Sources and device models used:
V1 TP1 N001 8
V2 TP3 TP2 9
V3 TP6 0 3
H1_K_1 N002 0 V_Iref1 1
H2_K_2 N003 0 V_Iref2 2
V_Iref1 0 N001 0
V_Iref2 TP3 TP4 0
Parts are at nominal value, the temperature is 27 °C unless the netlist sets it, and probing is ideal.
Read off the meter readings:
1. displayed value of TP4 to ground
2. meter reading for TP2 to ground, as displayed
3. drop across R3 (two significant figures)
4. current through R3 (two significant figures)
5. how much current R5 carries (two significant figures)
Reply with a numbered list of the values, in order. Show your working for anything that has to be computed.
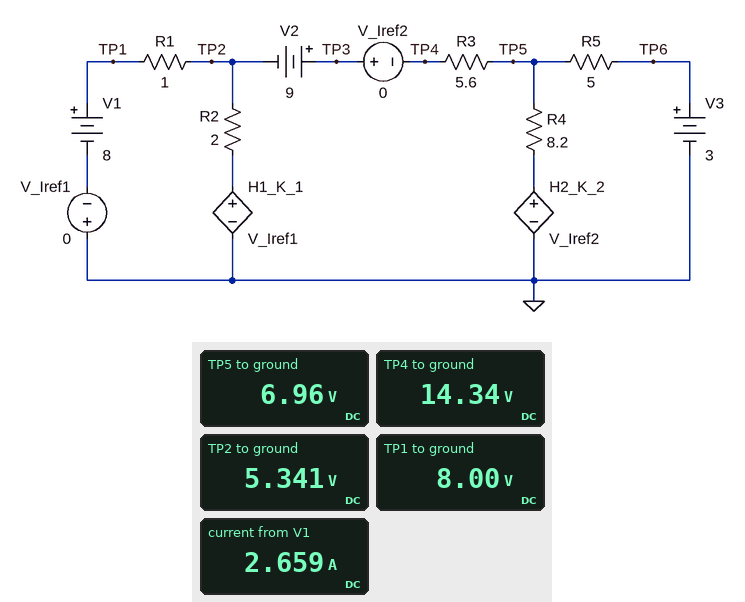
1. 14.34 V
2. 5.341 V
3. 14.34 V - 6.96 V = 7.4 V
4. (14.34 V - 6.96 V) / 5.6 Ω = 1.3 A
5. (6.96 V - 3 V) / 5 Ω = 790 mA
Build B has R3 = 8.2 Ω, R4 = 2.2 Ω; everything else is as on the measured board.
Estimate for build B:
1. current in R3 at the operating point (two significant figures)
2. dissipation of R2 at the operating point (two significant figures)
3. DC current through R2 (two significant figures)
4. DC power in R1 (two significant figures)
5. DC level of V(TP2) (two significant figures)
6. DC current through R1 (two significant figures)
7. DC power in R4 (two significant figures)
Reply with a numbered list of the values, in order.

1. 1.2 A
2. 3.9 W
3. 1.4 A
4. 6.8 W
5. 5.4 V
6. 2.6 A
7. 1.9 W
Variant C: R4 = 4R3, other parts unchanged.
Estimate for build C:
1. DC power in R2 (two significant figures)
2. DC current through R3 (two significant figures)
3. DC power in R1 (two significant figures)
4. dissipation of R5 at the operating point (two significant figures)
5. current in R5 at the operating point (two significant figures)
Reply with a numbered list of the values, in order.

1. 3.3 W
2. 1.4 A
3. 7.4 W
4. 2.1 W
5. 650 mA
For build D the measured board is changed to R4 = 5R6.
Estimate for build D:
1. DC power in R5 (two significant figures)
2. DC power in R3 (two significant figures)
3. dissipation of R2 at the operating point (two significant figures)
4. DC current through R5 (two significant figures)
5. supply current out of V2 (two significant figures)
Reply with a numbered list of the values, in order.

1. 2.5 W
2. 11 W
3. 3.4 W
4. 710 mA
5. 1.4 A
